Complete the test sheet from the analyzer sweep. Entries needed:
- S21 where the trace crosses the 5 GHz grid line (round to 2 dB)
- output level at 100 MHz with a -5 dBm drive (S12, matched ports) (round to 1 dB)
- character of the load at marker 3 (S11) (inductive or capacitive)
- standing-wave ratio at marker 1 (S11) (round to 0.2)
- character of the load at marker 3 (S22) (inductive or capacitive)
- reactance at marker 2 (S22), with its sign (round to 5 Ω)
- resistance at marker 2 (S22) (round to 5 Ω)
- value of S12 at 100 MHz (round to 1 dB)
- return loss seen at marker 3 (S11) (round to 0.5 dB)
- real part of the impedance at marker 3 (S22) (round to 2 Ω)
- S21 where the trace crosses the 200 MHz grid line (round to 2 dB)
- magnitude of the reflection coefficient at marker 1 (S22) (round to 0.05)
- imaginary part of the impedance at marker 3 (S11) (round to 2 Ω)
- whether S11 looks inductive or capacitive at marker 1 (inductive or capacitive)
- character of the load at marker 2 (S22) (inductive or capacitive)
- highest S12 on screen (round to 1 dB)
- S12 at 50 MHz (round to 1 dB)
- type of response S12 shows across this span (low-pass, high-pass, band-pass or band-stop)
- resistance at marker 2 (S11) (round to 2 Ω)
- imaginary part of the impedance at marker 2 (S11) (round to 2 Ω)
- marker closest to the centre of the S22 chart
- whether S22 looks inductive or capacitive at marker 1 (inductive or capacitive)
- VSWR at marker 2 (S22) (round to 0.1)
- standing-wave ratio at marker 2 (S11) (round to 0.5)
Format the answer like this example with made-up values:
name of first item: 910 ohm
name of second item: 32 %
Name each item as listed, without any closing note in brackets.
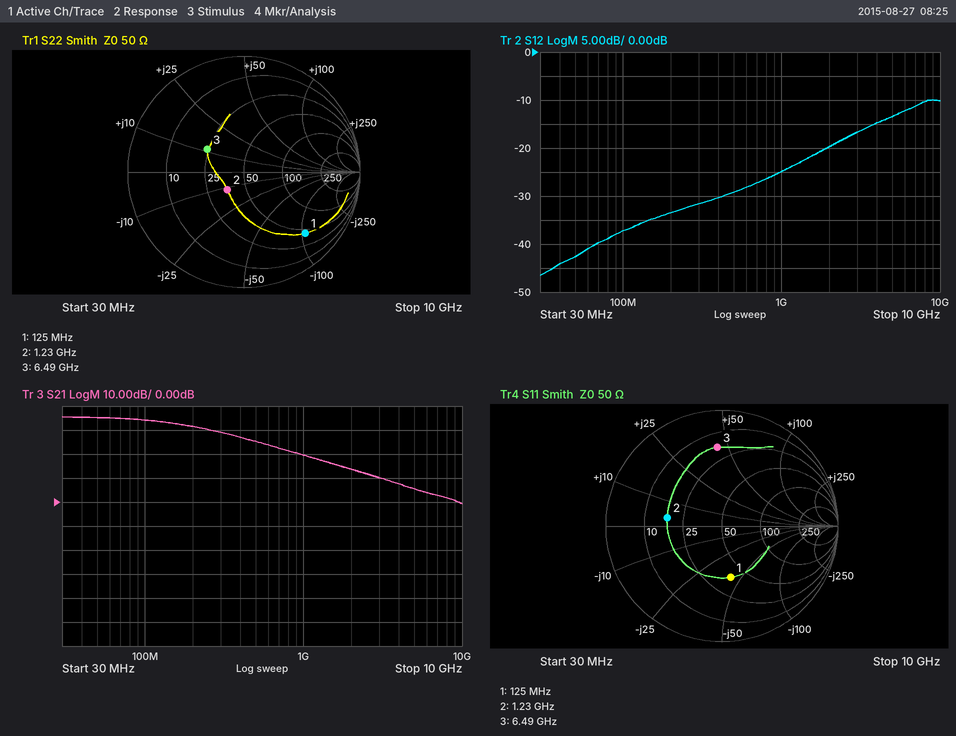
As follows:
S21 where the trace crosses the 5 GHz grid line: 6 dB
output level at 100 MHz with a -5 dBm drive (S12, matched ports): -42 dBm
character of the load at marker 3 (S11): inductive
standing-wave ratio at marker 1 (S11): 2.6
character of the load at marker 3 (S22): inductive
reactance at marker 2 (S22), with its sign: -10 Ω
resistance at marker 2 (S22): 35 Ω
value of S12 at 100 MHz: -37 dB
return loss seen at marker 3 (S11): 3.5 dB
real part of the impedance at marker 3 (S22): 24 Ω
S21 where the trace crosses the 200 MHz grid line: 32 dB
magnitude of the reflection coefficient at marker 1 (S22): 0.75
imaginary part of the impedance at marker 3 (S11): +44 Ω
whether S11 looks inductive or capacitive at marker 1: capacitive
character of the load at marker 2 (S22): capacitive
highest S12 on screen: -10 dB
S12 at 50 MHz: -43 dB
type of response S12 shows across this span: high-pass
resistance at marker 2 (S11): 18 Ω
imaginary part of the impedance at marker 2 (S11): +4 Ω
marker closest to the centre of the S22 chart: marker 2
whether S22 looks inductive or capacitive at marker 1: capacitive
VSWR at marker 2 (S22): 1.5
standing-wave ratio at marker 2 (S11): 3.0
